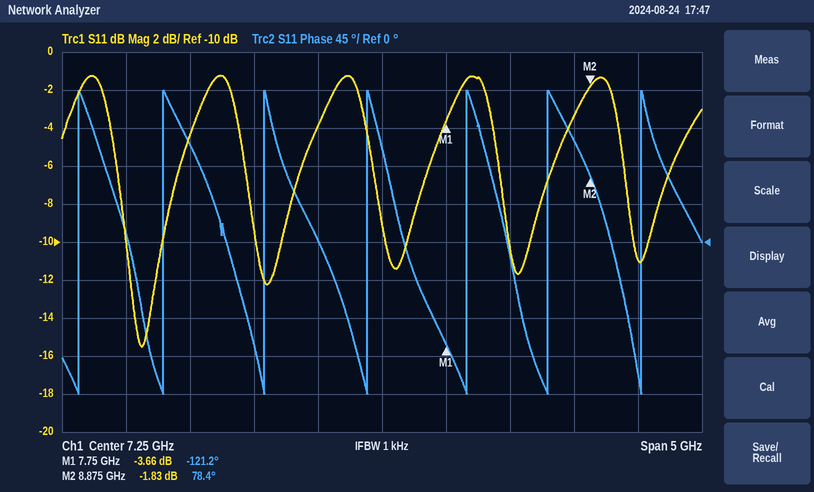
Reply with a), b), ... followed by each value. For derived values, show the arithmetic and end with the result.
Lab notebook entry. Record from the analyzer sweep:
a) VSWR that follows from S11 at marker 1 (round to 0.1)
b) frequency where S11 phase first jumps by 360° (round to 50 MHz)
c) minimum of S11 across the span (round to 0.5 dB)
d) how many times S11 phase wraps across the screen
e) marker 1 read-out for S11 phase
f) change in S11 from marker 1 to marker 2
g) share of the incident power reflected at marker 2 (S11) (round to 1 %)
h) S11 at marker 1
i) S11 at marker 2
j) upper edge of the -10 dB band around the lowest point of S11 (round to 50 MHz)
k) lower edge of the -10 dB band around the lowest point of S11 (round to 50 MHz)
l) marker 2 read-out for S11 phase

a) (1 + 0.6561)/(1 − 0.6561) ≈ 4.8
b) 4.90 GHz
c) -15.5 dB
d) 7
e) -121.2°
f) -1.83 − (-3.66) = 1.83 dB
g) 10^(-1.83/10) ≈ 66 %
h) -3.66 dB
i) -1.83 dB
j) 5.55 GHz
k) 5.25 GHz
l) 78.4°
